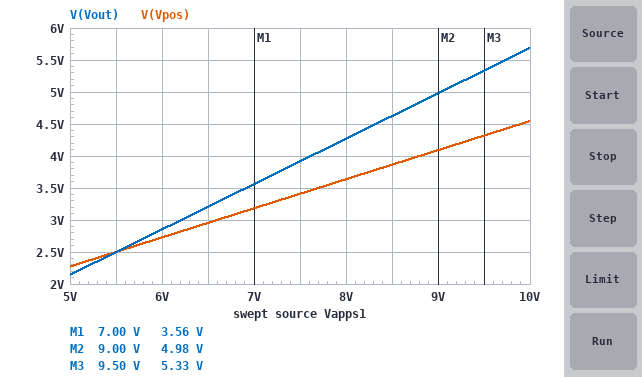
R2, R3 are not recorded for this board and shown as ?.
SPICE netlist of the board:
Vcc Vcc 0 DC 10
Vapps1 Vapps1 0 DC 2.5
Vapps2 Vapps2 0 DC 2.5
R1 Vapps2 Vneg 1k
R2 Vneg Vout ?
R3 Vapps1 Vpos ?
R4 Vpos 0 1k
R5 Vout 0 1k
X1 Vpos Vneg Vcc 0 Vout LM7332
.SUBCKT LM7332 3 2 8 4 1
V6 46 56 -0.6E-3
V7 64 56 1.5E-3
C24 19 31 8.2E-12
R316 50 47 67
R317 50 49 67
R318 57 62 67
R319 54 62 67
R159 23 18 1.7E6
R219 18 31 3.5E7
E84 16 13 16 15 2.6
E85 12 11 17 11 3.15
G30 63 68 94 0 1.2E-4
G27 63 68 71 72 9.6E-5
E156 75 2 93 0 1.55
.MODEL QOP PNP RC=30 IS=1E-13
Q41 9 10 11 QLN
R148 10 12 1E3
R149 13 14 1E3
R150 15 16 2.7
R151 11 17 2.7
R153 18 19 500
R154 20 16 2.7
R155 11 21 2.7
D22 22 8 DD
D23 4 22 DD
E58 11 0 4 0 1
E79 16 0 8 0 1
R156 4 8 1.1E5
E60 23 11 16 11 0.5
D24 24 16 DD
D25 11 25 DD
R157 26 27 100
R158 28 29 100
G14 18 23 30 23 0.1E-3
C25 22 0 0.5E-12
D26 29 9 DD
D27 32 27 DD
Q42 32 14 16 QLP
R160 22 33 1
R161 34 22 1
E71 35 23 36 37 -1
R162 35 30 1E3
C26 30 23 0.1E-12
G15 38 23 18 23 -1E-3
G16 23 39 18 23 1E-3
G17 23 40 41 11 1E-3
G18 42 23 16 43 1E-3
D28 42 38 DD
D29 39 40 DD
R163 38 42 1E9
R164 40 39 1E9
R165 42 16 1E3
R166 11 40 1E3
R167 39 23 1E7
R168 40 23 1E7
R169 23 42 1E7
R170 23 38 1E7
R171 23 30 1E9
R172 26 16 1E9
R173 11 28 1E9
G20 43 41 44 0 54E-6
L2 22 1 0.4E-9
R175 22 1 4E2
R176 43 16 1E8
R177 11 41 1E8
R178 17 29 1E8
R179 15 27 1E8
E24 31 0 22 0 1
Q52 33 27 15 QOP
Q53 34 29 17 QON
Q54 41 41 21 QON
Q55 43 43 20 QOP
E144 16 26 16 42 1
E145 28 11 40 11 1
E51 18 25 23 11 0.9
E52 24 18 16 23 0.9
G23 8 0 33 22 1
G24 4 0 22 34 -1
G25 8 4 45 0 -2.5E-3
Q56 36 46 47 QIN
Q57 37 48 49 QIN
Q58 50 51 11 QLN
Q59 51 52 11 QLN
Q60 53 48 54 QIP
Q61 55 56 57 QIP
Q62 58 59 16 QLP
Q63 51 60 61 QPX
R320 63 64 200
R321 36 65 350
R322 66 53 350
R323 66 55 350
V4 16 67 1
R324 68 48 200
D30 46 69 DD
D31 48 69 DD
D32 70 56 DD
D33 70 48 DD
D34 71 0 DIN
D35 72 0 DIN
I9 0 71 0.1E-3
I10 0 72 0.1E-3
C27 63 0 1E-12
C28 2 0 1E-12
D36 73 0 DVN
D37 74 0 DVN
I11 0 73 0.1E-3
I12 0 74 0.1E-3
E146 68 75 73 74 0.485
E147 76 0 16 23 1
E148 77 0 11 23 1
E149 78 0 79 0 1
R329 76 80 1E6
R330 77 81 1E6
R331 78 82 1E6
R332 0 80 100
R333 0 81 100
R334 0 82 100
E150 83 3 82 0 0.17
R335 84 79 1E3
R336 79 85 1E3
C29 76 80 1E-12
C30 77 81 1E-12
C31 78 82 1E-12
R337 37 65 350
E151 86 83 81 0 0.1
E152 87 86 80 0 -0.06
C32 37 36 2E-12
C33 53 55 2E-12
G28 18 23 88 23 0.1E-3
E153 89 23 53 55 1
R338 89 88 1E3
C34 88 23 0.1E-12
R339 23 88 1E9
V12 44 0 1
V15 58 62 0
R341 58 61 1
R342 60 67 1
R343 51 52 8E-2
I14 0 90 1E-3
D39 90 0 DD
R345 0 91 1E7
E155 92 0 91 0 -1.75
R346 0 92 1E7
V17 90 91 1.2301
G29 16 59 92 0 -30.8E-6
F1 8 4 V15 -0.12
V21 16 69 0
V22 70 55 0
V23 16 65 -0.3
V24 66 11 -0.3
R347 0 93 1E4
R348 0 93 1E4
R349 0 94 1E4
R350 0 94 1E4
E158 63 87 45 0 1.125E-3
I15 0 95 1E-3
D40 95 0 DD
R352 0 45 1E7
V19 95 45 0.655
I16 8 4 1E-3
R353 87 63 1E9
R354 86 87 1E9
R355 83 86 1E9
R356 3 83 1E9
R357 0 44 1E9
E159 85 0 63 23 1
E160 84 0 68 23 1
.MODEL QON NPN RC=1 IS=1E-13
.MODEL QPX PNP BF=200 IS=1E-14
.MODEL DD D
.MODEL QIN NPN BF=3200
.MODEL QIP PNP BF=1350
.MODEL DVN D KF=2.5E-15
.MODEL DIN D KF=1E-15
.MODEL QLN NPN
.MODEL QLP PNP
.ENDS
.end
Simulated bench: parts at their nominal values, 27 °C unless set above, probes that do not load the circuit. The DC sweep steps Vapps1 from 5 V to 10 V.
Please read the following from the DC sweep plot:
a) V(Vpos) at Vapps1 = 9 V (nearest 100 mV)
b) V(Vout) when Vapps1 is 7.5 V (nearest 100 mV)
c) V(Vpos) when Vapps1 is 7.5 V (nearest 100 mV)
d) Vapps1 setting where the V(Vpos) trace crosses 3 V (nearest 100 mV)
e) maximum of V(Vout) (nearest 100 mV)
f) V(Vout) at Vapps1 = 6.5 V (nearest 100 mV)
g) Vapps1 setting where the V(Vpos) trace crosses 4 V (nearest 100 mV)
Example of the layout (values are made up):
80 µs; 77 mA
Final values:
4.1 V; 3.9 V; 3.4 V; 6.6 V; 5.7 V; 3.2 V; 8.8 V
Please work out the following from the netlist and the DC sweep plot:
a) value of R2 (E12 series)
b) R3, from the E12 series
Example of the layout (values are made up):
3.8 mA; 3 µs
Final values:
560 Ω; 1.2 kΩ
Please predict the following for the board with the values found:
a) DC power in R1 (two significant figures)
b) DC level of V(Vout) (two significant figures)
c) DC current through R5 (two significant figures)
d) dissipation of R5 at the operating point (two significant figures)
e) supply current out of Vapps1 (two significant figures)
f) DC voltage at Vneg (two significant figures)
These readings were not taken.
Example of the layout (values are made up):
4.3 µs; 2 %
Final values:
1.9 mW; 370 mV; 370 µA; 140 µW; 1.1 mA; 1.1 V
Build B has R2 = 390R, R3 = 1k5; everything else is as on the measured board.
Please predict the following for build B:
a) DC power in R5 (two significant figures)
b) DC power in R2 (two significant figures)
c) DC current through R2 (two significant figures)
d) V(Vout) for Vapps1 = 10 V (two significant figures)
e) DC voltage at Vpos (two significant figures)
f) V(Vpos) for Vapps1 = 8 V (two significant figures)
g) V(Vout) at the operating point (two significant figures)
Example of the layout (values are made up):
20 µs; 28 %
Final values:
170 µW; 880 µW; 1.5 mA; 4.6 V; 1.0 V; 3.2 V; 410 mV
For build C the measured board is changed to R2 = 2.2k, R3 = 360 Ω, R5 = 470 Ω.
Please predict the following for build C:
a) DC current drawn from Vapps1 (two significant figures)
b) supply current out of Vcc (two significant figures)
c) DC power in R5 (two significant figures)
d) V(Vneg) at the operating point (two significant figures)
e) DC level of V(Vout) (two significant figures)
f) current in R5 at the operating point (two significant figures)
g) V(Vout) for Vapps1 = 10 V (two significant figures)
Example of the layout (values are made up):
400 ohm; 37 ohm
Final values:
1.8 mA; 910 µA; 300 µW; 1.8 V; 380 mV; 800 µA; 9.2 V
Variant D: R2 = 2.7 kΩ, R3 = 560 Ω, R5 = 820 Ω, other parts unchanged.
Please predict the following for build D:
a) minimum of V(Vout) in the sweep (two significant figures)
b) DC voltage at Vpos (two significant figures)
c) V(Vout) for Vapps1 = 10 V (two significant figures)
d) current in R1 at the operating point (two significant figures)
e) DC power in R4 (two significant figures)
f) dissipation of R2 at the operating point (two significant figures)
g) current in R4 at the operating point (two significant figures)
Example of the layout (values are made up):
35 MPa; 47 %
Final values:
5.1 V; 1.6 V; 9.5 V; 660 µA; 2.6 mW; 1.2 mW; 1.6 mA
